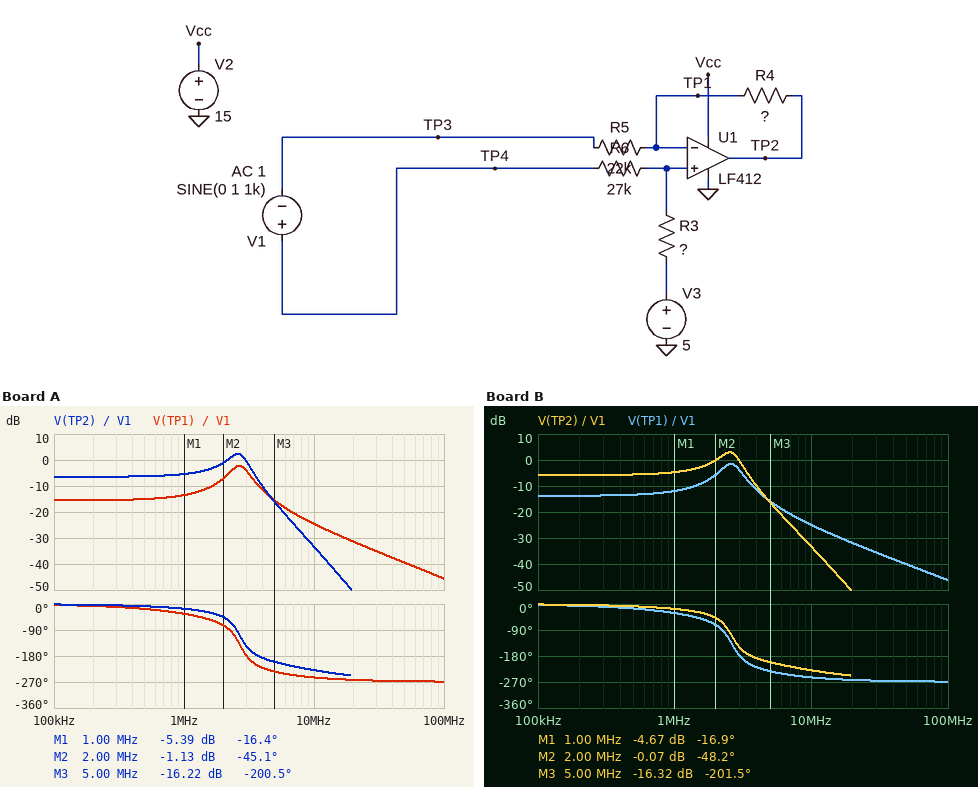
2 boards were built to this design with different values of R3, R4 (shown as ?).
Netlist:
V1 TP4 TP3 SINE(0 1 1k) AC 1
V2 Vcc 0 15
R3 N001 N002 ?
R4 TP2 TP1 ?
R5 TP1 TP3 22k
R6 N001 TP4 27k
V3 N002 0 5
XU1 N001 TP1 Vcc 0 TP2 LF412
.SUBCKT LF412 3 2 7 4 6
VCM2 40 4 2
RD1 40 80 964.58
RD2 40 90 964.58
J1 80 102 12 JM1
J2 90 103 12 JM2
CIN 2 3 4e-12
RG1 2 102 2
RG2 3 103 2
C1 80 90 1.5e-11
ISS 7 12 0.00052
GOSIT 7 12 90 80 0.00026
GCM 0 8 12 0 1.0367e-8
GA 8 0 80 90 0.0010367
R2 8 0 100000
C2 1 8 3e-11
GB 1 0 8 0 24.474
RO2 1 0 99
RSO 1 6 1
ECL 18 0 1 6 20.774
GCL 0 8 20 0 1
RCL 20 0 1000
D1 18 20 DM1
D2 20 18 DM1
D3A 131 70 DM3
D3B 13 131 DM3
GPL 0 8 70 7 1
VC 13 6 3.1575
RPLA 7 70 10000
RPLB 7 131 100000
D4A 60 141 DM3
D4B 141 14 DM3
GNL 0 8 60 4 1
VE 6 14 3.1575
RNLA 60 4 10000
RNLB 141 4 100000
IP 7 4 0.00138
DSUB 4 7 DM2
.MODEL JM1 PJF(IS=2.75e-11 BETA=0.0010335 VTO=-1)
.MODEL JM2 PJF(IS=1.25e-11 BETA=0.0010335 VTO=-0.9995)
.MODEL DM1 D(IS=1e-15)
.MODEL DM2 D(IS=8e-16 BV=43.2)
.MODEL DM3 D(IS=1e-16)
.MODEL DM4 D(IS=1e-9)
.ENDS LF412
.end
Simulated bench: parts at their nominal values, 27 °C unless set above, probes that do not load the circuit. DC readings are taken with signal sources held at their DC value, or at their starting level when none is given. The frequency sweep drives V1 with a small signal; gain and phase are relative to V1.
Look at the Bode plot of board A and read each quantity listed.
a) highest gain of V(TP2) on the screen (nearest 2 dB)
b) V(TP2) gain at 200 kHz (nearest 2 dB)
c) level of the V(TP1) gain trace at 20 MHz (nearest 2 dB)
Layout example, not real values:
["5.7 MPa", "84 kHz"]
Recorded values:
["2 dB", "-6 dB", "-32 dB"]
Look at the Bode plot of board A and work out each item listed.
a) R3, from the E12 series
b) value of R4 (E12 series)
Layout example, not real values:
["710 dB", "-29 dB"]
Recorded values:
["8.2 kΩ", "15 kΩ"]
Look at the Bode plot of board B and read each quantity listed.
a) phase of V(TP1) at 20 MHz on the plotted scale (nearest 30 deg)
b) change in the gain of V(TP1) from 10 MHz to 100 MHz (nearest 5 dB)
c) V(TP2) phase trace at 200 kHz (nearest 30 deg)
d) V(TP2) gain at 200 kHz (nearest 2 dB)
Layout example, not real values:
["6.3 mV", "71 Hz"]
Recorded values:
["-270 deg", "-20 dB", "0 deg", "-6 dB"]
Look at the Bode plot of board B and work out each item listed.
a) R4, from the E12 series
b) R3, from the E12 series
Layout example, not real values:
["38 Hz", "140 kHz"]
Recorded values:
["15 kΩ", "10 kΩ"]
